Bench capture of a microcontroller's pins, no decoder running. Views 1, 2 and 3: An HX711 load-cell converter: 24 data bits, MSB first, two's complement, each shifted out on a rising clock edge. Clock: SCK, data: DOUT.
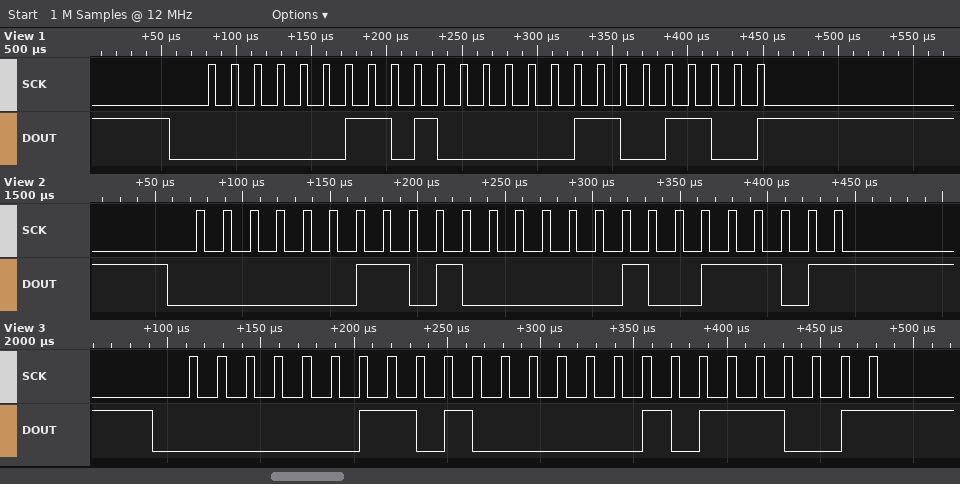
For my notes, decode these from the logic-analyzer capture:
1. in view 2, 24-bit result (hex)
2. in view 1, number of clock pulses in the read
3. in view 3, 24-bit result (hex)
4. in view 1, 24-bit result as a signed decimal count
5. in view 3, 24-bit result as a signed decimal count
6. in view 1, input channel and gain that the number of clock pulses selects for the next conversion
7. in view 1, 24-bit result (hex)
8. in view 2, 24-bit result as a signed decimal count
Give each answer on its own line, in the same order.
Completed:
0x03409D
25
0x0340B9
213196
213177
channel A, gain 128
0x0340CC
213149
